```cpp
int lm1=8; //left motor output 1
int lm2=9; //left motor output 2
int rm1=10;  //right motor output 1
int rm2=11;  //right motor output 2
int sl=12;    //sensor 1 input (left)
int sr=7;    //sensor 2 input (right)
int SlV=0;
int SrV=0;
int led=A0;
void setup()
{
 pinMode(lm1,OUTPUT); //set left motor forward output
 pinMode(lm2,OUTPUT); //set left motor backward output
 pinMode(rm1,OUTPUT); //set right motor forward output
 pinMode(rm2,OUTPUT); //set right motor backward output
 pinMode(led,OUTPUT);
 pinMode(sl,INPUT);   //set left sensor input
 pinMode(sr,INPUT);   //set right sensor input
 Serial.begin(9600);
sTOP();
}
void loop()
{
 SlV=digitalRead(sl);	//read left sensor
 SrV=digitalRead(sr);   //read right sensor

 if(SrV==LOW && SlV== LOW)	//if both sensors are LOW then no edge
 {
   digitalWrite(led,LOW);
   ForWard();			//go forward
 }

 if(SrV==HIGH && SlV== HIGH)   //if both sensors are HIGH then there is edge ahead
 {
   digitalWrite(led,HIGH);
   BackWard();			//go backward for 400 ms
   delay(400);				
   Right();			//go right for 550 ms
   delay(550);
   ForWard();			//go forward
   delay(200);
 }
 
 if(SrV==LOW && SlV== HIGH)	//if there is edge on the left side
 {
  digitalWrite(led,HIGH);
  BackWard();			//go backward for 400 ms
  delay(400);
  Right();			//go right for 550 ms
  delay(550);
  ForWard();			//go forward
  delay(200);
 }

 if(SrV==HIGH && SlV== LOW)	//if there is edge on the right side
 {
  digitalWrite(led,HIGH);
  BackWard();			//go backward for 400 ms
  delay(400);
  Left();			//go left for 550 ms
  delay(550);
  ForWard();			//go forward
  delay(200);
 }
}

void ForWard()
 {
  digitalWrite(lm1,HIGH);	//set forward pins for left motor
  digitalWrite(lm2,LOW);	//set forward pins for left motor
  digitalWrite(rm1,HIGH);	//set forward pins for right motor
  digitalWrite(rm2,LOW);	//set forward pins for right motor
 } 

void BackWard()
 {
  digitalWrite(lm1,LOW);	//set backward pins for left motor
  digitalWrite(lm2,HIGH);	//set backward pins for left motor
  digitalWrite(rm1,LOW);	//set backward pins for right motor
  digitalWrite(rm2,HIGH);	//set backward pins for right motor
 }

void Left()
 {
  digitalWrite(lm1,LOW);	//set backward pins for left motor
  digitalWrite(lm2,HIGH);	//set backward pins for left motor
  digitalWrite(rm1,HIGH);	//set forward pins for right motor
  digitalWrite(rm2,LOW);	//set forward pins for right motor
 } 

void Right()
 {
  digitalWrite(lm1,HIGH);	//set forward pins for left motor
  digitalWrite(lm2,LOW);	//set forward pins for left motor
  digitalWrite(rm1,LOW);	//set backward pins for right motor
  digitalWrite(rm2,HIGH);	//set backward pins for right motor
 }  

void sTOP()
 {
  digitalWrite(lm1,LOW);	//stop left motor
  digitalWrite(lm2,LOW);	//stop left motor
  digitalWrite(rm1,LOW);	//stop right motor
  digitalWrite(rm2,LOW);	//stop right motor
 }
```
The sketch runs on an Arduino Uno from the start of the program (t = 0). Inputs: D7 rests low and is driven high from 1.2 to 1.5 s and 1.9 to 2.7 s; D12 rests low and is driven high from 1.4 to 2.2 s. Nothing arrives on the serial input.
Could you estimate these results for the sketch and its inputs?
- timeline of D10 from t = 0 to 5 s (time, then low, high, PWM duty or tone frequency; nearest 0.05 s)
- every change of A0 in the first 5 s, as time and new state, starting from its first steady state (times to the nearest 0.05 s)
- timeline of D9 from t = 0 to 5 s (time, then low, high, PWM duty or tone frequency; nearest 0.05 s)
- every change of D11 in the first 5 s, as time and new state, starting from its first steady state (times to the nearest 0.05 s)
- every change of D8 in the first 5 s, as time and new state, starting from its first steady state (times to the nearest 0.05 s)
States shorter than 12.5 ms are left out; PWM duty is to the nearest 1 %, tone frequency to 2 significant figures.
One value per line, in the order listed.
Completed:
0 s high; 1.2 s low; 1.6 s high; 2.35 s low; 2.75 s high
0 s low; 1.2 s high; 3.5 s low
0 s low; 1.2 s high; 2.15 s low; 2.35 s high; 3.3 s low
0 s low; 1.2 s high; 1.6 s low; 2.35 s high; 2.75 s low
0 s high; 1.2 s low; 2.15 s high; 2.35 s low; 3.3 s high
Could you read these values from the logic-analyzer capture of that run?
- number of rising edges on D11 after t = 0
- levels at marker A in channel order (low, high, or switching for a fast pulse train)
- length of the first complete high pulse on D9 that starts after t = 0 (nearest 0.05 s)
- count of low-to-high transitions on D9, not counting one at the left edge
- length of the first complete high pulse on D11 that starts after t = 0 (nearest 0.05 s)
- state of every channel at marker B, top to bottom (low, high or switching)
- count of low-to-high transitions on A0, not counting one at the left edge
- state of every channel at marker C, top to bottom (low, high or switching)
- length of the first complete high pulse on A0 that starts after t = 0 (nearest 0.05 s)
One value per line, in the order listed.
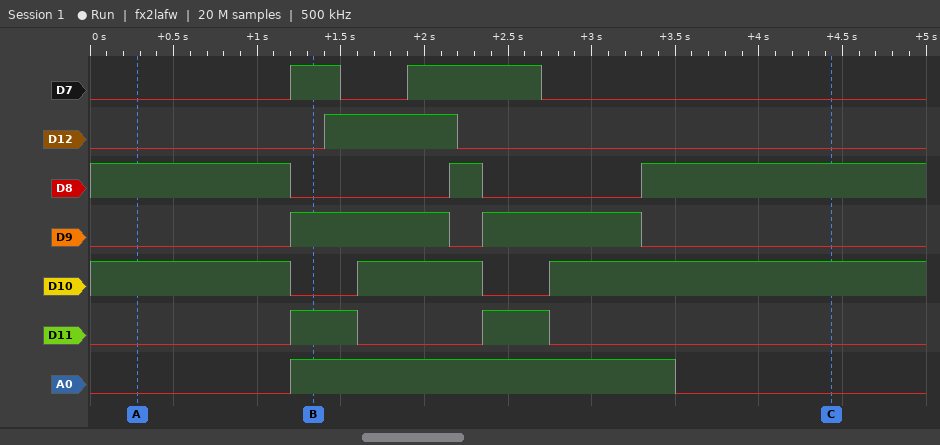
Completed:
2
D7 low, D12 low, D8 high, D9 low, D10 high, D11 low, A0 low
0.95 s
2
0.40 s
D7 high, D12 low, D8 low, D9 high, D10 low, D11 high, A0 high
1
D7 low, D12 low, D8 high, D9 low, D10 high, D11 low, A0 low
2.30 s
